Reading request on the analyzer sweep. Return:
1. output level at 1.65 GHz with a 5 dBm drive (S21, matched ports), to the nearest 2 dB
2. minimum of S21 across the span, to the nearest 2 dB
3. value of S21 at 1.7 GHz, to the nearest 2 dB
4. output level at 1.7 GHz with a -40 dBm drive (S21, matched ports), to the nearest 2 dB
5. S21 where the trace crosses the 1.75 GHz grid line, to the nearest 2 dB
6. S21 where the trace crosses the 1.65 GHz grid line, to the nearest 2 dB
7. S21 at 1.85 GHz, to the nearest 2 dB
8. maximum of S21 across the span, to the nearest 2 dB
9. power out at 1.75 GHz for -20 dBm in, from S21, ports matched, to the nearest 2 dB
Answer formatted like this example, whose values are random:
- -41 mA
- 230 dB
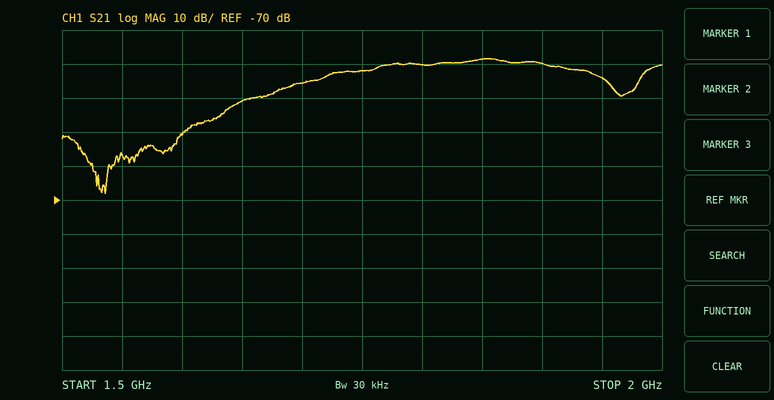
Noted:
- -36 dBm
- -68 dB
- -36 dB
- -76 dBm
- -32 dB
- -40 dB
- -28 dB
- -28 dB
- -52 dBm
